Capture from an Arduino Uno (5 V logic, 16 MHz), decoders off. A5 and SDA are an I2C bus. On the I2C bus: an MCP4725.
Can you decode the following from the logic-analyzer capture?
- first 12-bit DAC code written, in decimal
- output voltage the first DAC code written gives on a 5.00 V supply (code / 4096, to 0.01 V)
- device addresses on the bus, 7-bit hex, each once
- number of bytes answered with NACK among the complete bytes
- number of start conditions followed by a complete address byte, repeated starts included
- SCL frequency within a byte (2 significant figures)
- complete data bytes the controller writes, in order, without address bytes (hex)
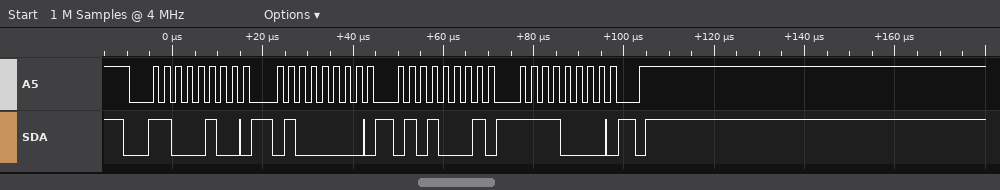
1311
1.60 V
0x62
0
1
400 kHz
40 51 F0
